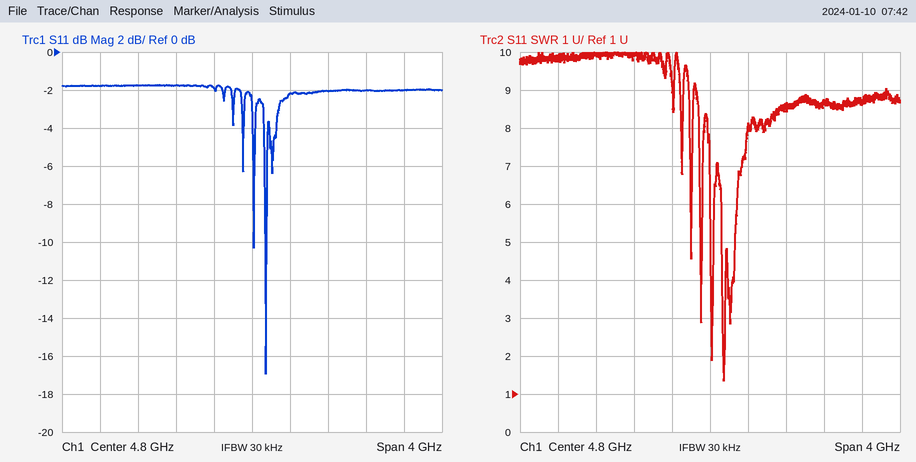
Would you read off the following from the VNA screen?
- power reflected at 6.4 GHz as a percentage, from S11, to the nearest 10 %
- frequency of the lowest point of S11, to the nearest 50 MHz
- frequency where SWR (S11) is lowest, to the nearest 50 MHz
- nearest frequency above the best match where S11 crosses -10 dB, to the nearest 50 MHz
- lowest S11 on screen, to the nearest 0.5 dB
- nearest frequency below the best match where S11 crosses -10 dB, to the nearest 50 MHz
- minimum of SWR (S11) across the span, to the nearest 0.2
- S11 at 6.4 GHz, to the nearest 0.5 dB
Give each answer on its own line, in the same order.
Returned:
60 %
4.95 GHz
4.95 GHz
4.95 GHz
-17.0 dB
4.95 GHz
1.4
-2.0 dB
